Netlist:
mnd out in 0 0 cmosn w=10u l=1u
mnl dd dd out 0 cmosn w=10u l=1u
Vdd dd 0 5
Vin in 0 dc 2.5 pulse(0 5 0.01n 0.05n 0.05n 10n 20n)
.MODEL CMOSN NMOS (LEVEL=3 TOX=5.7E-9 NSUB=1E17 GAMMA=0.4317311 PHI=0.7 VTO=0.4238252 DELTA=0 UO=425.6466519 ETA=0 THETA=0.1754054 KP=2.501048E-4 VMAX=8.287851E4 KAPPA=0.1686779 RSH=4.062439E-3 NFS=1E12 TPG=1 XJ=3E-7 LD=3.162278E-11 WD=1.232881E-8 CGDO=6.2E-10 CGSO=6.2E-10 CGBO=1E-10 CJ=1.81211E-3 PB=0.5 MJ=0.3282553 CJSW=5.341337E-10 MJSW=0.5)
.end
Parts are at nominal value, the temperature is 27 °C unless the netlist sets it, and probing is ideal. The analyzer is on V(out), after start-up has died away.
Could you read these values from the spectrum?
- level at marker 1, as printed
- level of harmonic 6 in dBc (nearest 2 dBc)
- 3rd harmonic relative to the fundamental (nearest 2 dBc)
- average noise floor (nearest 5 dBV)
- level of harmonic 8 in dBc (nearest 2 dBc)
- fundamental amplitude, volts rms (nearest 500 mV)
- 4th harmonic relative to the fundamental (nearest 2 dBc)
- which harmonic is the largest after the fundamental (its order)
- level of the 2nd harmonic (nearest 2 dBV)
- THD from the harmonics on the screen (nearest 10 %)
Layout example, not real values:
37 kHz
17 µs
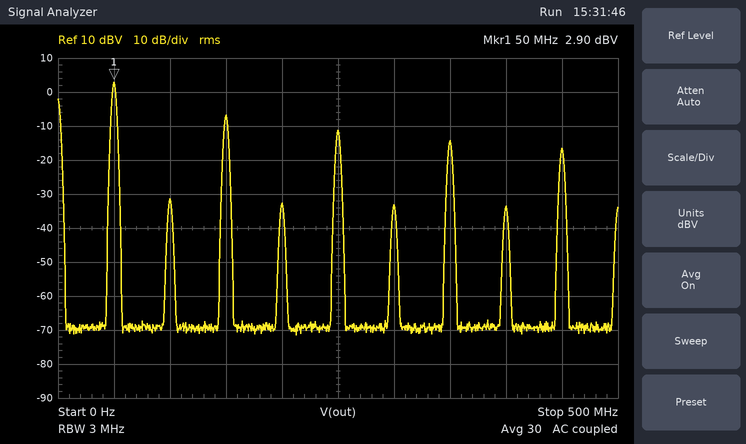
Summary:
2.90 dBV
-36 dBc
-10 dBc
-70 dBV
-36 dBc
1.5 V
-36 dBc
3
-32 dBV
40 %
